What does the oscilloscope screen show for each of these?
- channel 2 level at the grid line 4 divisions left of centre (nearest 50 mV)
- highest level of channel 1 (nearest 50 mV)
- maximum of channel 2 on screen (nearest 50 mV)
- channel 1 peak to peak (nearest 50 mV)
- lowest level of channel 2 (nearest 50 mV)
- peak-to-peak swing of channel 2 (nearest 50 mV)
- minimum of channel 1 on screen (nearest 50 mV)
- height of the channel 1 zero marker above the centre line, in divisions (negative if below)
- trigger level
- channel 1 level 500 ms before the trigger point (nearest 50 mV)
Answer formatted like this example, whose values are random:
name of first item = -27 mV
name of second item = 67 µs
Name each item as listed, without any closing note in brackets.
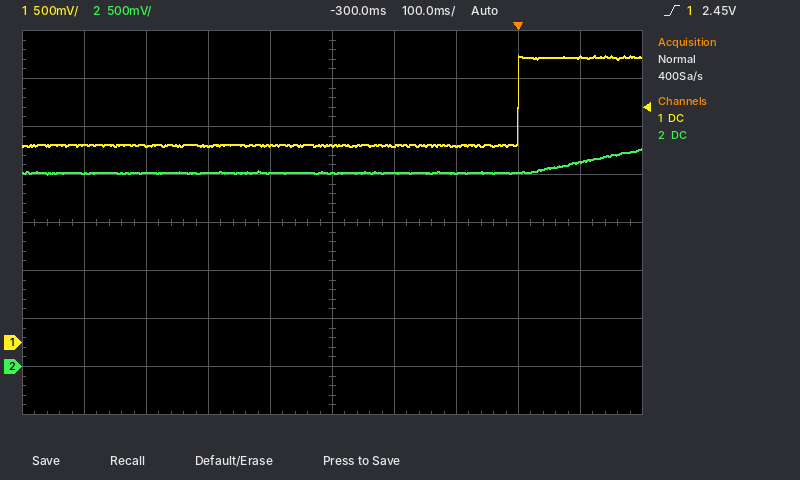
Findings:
channel 2 level at the grid line 4 divisions left of centre = 2.00 V
highest level of channel 1 = 3.00 V
maximum of channel 2 on screen = 2.25 V
channel 1 peak to peak = 950 mV
lowest level of channel 2 = 2.00 V
peak-to-peak swing of channel 2 = 250 mV
minimum of channel 1 on screen = 2.05 V
height of the channel 1 zero marker above the centre line, in divisions = -2.5 div
trigger level = 2.45 V
channel 1 level 500 ms before the trigger point = 2.05 V
